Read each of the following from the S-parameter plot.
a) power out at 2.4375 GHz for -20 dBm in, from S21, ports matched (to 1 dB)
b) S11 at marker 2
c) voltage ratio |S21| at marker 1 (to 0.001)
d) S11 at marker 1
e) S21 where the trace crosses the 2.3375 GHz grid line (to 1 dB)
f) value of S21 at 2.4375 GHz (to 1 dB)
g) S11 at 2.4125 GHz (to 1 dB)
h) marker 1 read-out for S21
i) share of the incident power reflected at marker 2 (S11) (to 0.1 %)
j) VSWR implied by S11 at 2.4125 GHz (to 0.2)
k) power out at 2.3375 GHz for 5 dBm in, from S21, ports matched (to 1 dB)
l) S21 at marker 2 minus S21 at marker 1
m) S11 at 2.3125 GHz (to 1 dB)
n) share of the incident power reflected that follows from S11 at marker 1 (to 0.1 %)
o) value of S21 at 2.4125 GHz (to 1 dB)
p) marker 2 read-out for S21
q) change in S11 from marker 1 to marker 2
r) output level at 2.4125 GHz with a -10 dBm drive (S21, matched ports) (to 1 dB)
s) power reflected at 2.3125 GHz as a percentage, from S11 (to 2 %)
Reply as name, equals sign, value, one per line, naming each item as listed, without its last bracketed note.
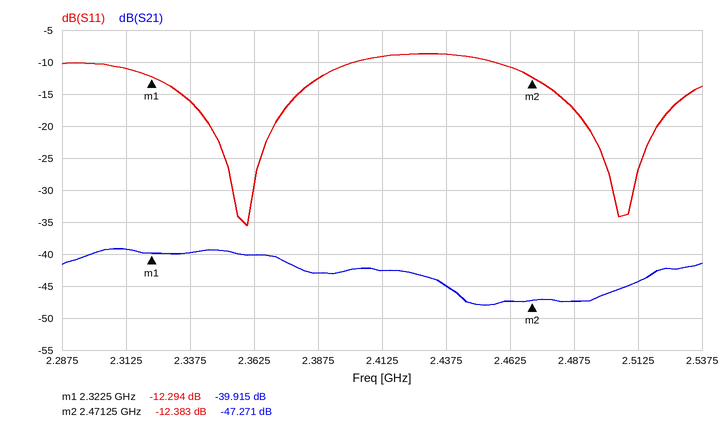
power out at 2.4375 GHz for -20 dBm in, from S21, ports matched = -65 dBm
S11 at marker 2 = -12.383 dB
voltage ratio |S21| at marker 1 = 0.010
S11 at marker 1 = -12.294 dB
S21 where the trace crosses the 2.3375 GHz grid line = -40 dB
value of S21 at 2.4375 GHz = -45 dB
S11 at 2.4125 GHz = -9 dB
marker 1 read-out for S21 = -39.915 dB
share of the incident power reflected at marker 2 (S11) = 5.8 %
VSWR implied by S11 at 2.4125 GHz = 2.0
power out at 2.3375 GHz for 5 dBm in, from S21, ports matched = -35 dBm
S21 at marker 2 minus S21 at marker 1 = -7.356 dB
S11 at 2.3125 GHz = -11 dB
share of the incident power reflected that follows from S11 at marker 1 = 5.9 %
value of S21 at 2.4125 GHz = -43 dB
marker 2 read-out for S21 = -47.271 dB
change in S11 from marker 1 to marker 2 = -0.089 dB
output level at 2.4125 GHz with a -10 dBm drive (S21, matched ports) = -53 dBm
power reflected at 2.3125 GHz as a percentage, from S11 = 8 %
